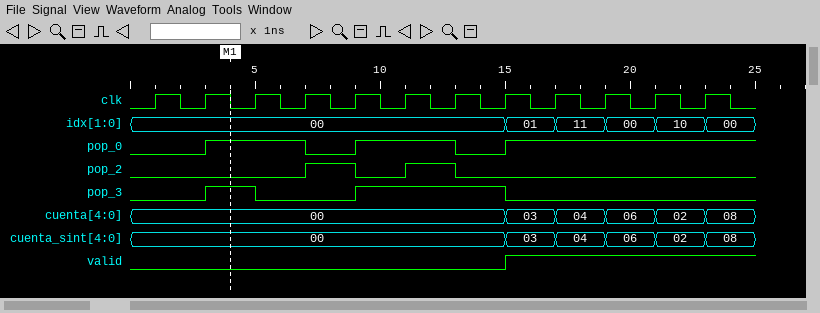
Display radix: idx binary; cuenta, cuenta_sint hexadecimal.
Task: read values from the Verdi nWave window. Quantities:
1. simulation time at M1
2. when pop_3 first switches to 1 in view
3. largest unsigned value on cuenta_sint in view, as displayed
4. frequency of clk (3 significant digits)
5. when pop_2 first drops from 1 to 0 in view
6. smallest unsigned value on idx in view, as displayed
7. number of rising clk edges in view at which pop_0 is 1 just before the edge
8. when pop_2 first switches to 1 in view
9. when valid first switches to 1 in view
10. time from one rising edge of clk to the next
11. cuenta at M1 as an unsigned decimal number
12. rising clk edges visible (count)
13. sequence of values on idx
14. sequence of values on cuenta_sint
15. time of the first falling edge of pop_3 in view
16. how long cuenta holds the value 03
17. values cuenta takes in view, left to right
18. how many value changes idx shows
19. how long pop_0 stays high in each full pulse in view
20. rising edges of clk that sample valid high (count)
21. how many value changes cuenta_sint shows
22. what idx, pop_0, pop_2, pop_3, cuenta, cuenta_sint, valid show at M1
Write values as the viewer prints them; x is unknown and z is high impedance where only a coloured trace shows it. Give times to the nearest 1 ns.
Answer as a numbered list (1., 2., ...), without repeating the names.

1. 4 ns
2. 3 ns
3. 08
4. 500 MHz
5. 9 ns
6. 00
7. 8
8. 7 ns
9. 15 ns
10. 2 ns
11. 0
12. 12
13. 00, 01, 11, 00, 10, 00
14. 00, 03, 04, 06, 02, 08
15. 5 ns
16. 2 ns
17. 00, 03, 04, 06, 02, 08
18. 5
19. 4 ns, 4 ns
20. 4
21. 5
22. idx=00, pop_0=1, pop_2=0, pop_3=1, cuenta=00, cuenta_sint=00, valid=0
